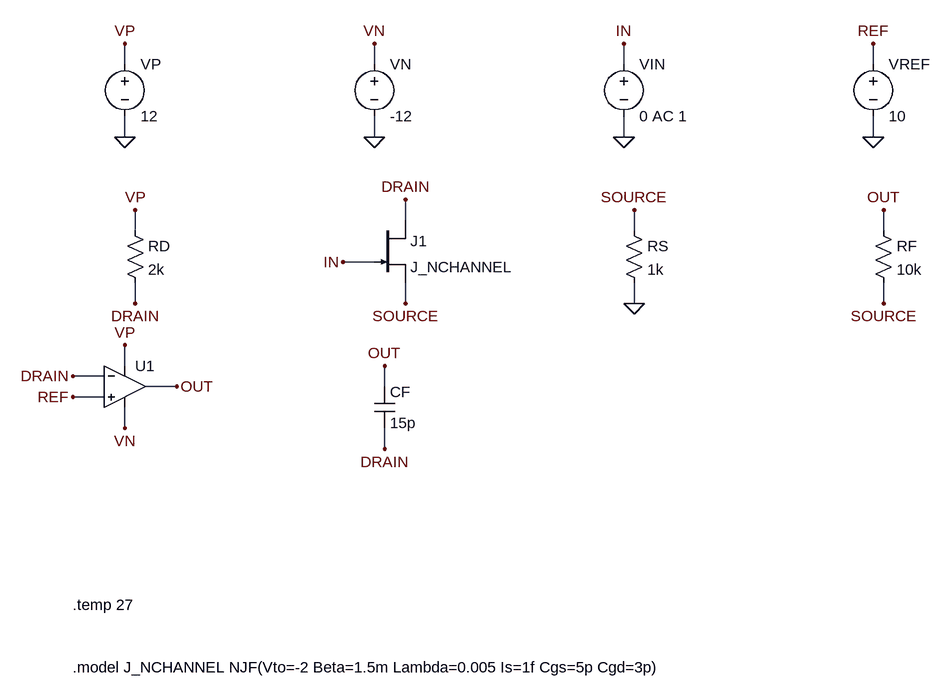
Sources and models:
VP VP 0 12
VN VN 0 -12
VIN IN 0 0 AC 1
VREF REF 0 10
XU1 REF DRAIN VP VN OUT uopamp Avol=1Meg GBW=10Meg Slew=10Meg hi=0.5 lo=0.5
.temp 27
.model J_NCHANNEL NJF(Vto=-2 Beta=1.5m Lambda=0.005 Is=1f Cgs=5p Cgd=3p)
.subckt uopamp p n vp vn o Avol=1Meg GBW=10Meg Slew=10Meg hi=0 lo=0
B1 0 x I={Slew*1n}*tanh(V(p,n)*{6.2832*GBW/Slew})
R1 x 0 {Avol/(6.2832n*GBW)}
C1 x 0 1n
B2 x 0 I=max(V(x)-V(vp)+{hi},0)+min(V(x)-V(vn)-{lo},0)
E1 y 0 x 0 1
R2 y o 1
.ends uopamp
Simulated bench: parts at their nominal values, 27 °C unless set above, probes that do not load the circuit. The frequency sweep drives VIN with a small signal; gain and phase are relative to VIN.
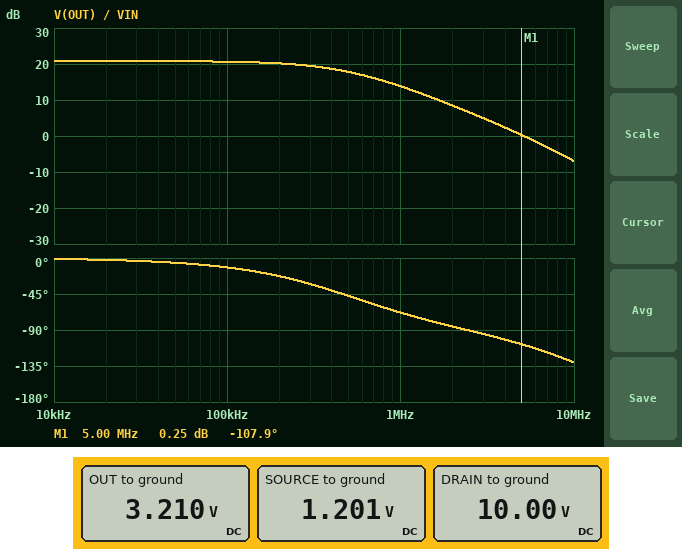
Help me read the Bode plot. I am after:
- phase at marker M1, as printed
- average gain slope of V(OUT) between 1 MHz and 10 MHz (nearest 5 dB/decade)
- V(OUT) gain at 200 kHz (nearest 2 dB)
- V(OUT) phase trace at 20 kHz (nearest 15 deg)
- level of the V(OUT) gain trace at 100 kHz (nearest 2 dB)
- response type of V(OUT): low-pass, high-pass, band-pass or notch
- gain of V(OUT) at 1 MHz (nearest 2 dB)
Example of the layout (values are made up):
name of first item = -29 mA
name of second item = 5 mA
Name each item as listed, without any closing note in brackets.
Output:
phase at marker M1, as printed = -107.9 deg
average gain slope of V(OUT) between 1 MHz and 10 MHz = -20 dB/decade
V(OUT) gain at 200 kHz = 20 dB
V(OUT) phase trace at 20 kHz = 0 deg
level of the V(OUT) gain trace at 100 kHz = 20 dB
response type of V(OUT): low-pass, high-pass, band-pass or notch = low-pass
gain of V(OUT) at 1 MHz = 14 dB
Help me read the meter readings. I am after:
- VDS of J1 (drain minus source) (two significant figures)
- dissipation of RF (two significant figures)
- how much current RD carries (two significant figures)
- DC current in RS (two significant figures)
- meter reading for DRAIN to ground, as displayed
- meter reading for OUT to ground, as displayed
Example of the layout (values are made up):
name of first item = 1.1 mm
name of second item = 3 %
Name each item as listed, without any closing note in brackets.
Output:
VDS of J1 (drain minus source) = 8.8 V
dissipation of RF = 400 µW
how much current RD carries = 1.0 mA
DC current in RS = 1.2 mA
meter reading for DRAIN to ground, as displayed = 10.00 V
meter reading for OUT to ground, as displayed = 3.210 V
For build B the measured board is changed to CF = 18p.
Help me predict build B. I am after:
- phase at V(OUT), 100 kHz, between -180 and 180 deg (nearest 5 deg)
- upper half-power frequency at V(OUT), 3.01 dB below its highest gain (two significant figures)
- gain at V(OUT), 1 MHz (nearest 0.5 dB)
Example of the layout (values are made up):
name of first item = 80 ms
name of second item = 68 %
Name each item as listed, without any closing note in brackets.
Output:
phase at V(OUT), 100 kHz, between -180 and 180 deg = -15 deg
upper half-power frequency at V(OUT), 3.01 dB below its highest gain = 440 kHz
gain at V(OUT), 1 MHz = 13.0 dB
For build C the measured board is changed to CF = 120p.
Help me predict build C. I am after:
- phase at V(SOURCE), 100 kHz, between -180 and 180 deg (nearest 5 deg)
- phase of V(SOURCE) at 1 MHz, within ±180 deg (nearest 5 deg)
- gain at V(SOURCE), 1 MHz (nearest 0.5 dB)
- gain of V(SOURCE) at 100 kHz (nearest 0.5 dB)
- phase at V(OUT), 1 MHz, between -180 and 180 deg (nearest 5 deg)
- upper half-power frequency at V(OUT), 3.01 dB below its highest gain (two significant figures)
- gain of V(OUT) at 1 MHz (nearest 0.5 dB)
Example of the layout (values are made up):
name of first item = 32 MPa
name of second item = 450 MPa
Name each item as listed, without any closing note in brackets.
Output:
phase at V(SOURCE), 100 kHz, between -180 and 180 deg = -10 deg
phase of V(SOURCE) at 1 MHz, within ±180 deg = 0 deg
gain at V(SOURCE), 1 MHz = -3.0 dB
gain of V(SOURCE) at 100 kHz = -1.5 dB
phase at V(OUT), 1 MHz, between -180 and 180 deg = -90 deg
upper half-power frequency at V(OUT), 3.01 dB below its highest gain = 87 kHz
gain of V(OUT) at 1 MHz = -0.5 dB
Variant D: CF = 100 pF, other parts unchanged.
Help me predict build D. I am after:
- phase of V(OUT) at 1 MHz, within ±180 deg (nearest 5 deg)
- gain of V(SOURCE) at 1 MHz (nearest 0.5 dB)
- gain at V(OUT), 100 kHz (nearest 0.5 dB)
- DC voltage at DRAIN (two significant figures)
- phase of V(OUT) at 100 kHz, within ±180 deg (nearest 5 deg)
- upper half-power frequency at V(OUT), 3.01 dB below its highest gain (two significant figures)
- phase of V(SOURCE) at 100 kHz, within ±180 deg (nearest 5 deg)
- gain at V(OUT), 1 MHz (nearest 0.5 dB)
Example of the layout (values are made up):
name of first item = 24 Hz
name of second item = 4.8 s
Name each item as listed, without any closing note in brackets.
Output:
phase of V(OUT) at 1 MHz, within ±180 deg = -90 deg
gain of V(SOURCE) at 1 MHz = -3.0 dB
gain at V(OUT), 100 kHz = 18.0 dB
DC voltage at DRAIN = 10 V
phase of V(OUT) at 100 kHz, within ±180 deg = -45 deg
upper half-power frequency at V(OUT), 3.01 dB below its highest gain = 100 kHz
phase of V(SOURCE) at 100 kHz, within ±180 deg = -10 deg
gain at V(OUT), 1 MHz = 1.0 dB
